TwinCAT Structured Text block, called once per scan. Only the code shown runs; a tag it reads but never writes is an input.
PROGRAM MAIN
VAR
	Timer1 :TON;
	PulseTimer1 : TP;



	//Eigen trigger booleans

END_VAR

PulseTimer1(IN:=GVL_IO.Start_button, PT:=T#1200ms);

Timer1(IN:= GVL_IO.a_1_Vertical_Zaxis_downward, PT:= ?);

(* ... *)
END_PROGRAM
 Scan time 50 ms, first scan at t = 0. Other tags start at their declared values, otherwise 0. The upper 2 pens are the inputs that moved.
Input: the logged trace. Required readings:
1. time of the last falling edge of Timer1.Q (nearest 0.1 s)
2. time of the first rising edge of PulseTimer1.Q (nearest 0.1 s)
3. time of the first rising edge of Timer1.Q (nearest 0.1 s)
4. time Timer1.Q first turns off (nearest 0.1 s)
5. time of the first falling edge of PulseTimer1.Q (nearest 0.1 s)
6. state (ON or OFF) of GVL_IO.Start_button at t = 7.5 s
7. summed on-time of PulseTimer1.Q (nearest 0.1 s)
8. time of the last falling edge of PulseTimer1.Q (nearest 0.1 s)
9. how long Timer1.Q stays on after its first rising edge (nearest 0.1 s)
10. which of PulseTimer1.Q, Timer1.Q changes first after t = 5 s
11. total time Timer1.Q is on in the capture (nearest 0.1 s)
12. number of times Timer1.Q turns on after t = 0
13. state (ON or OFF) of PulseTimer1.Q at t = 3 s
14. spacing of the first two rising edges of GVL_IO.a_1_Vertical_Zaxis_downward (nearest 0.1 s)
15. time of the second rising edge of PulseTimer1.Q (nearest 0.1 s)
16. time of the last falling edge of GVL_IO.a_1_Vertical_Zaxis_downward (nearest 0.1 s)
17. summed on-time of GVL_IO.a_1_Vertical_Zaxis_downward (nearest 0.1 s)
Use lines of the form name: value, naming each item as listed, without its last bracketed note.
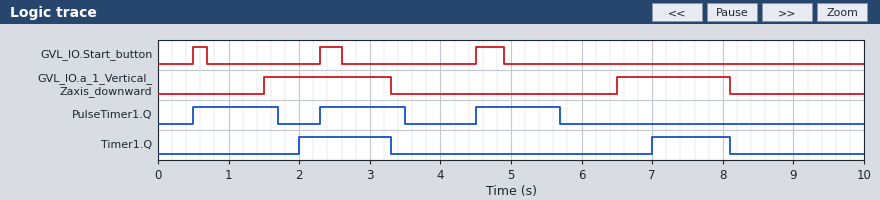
time of the last falling edge of Timer1.Q: 8.1 s
time of the first rising edge of PulseTimer1.Q: 0.5 s
time of the first rising edge of Timer1.Q: 2.0 s
time Timer1.Q first turns off: 3.3 s
time of the first falling edge of PulseTimer1.Q: 1.7 s
state (ON or OFF) of GVL_IO.Start_button at t = 7.5 s: OFF
summed on-time of PulseTimer1.Q: 3.6 s
time of the last falling edge of PulseTimer1.Q: 5.7 s
how long Timer1.Q stays on after its first rising edge: 1.3 s
which of PulseTimer1.Q, Timer1.Q changes first after t = 5 s: PulseTimer1.Q
total time Timer1.Q is on in the capture: 2.4 s
number of times Timer1.Q turns on after t = 0: 2
state (ON or OFF) of PulseTimer1.Q at t = 3 s: ON
spacing of the first two rising edges of GVL_IO.a_1_Vertical_Zaxis_downward: 5.0 s
time of the second rising edge of PulseTimer1.Q: 2.3 s
time of the last falling edge of GVL_IO.a_1_Vertical_Zaxis_downward: 8.1 s
summed on-time of GVL_IO.a_1_Vertical_Zaxis_downward: 3.4 s
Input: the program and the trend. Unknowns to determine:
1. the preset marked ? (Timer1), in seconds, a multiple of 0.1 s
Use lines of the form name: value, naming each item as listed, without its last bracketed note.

the preset marked ? (Timer1), in seconds, a multiple of 0.1 s: 0.5 s
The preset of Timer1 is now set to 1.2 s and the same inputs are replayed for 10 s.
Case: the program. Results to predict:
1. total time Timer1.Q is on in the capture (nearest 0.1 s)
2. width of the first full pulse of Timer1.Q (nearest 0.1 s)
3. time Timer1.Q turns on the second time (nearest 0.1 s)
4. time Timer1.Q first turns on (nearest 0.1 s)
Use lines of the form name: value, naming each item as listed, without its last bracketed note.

total time Timer1.Q is on in the capture: 1.0 s
width of the first full pulse of Timer1.Q: 0.6 s
time Timer1.Q turns on the second time: 7.7 s
time Timer1.Q first turns on: 2.7 s
